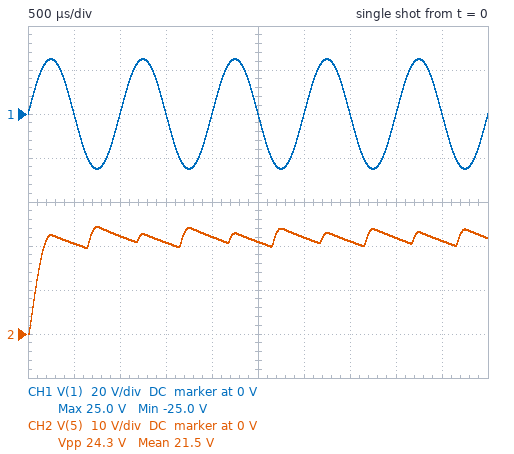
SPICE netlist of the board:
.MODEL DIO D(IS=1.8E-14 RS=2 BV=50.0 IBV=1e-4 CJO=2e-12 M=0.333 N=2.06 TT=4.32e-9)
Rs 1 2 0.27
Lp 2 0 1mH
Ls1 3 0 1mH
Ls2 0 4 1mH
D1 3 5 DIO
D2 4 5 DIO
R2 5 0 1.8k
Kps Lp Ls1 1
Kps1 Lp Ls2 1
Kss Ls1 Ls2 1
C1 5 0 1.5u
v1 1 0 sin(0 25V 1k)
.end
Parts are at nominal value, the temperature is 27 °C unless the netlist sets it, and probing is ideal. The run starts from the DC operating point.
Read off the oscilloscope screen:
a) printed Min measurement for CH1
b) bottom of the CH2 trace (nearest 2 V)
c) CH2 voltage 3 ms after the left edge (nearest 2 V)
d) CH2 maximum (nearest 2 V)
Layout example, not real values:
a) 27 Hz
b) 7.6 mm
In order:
a) -25.0 V
b) 0 V
c) 22 V
d) 24 V
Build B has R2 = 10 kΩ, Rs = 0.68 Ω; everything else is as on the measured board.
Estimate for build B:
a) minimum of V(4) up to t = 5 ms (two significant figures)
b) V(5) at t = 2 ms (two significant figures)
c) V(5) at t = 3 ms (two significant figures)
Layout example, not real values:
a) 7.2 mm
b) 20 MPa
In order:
a) -25 V
b) 24 V
c) 23 V
